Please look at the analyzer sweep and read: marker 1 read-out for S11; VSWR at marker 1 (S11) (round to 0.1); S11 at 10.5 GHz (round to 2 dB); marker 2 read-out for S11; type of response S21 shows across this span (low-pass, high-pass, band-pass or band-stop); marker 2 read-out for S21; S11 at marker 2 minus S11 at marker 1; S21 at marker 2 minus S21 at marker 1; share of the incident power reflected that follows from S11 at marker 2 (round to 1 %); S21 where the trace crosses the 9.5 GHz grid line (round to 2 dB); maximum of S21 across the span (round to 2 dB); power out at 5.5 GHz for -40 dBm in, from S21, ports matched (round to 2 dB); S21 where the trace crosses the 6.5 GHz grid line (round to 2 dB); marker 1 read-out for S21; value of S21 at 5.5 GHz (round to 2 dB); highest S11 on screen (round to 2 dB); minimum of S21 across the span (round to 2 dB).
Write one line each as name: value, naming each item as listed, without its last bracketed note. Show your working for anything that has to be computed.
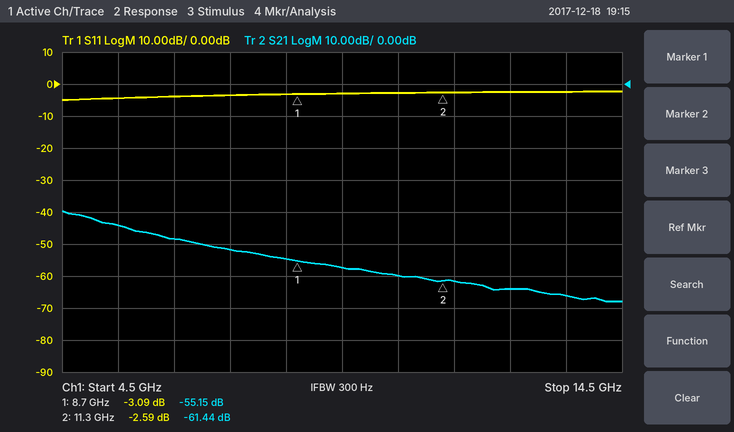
marker 1 read-out for S11: -3.09 dB
VSWR at marker 1 (S11): (1 + 0.7006)/(1 − 0.7006) ≈ 5.7
S11 at 10.5 GHz: -2 dB
marker 2 read-out for S11: -2.59 dB
type of response S21 shows across this span: low-pass
marker 2 read-out for S21: -61.44 dB
S11 at marker 2 minus S11 at marker 1: -2.59 − (-3.09) = 0.50 dB
S21 at marker 2 minus S21 at marker 1: -61.44 − (-55.15) = -6.29 dB
share of the incident power reflected that follows from S11 at marker 2: 10^(-2.59/10) ≈ 55 %
S21 where the trace crosses the 9.5 GHz grid line: -58 dB
maximum of S21 across the span: -40 dB
power out at 5.5 GHz for -40 dBm in, from S21, ports matched: -40 dBm + (-44 dB) = -84 dBm
S21 where the trace crosses the 6.5 GHz grid line: -48 dB
marker 1 read-out for S21: -55.15 dB
value of S21 at 5.5 GHz: -44 dB
highest S11 on screen: -2 dB
minimum of S21 across the span: -68 dB
